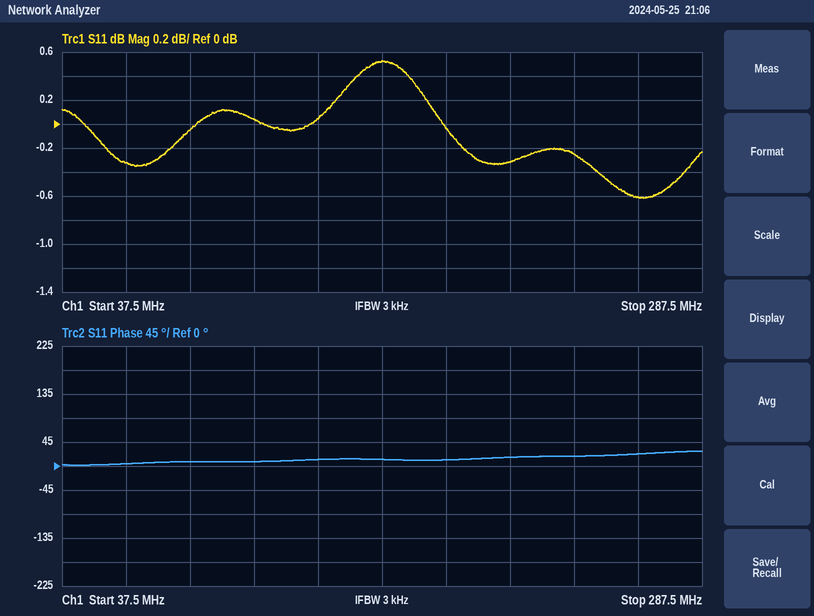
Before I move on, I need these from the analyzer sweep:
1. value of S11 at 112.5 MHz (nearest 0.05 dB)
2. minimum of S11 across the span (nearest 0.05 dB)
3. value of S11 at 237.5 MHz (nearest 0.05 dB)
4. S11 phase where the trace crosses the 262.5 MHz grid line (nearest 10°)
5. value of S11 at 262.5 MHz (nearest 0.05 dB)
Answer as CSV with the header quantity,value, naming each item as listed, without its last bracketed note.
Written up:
quantity,value
value of S11 at 112.5 MHz,0.05 dB
minimum of S11 across the span,-0.60 dB
value of S11 at 237.5 MHz,-0.25 dB
S11 phase where the trace crosses the 262.5 MHz grid line,20°
value of S11 at 262.5 MHz,-0.60 dB
